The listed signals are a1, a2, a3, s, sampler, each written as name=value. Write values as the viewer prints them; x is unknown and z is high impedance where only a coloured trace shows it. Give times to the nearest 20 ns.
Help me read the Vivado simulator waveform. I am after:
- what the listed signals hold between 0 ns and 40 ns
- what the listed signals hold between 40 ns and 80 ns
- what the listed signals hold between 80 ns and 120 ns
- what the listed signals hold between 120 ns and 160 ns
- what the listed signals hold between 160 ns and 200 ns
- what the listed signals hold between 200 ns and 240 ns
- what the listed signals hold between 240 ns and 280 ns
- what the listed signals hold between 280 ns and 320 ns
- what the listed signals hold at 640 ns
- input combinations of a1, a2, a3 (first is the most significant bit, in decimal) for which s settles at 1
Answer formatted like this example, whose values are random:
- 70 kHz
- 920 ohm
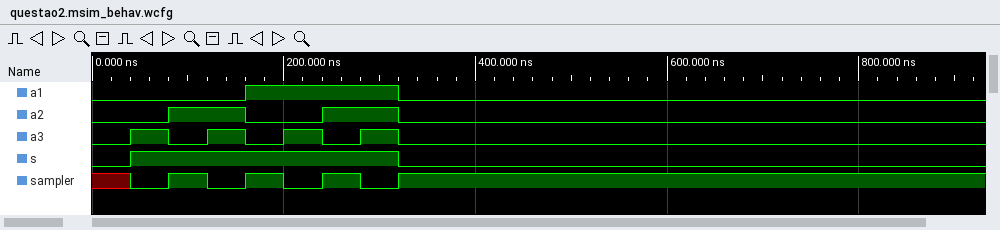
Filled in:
- a1=0, a2=0, a3=0, s=0, sampler=x
- a1=0, a2=0, a3=1, s=1, sampler=0
- a1=0, a2=1, a3=0, s=1, sampler=1
- a1=0, a2=1, a3=1, s=1, sampler=0
- a1=1, a2=0, a3=0, s=1, sampler=1
- a1=1, a2=0, a3=1, s=1, sampler=0
- a1=1, a2=1, a3=0, s=1, sampler=1
- a1=1, a2=1, a3=1, s=1, sampler=0
- a1=0, a2=0, a3=0, s=0, sampler=1
- 1, 2, 3, 4, 5, 6, 7
